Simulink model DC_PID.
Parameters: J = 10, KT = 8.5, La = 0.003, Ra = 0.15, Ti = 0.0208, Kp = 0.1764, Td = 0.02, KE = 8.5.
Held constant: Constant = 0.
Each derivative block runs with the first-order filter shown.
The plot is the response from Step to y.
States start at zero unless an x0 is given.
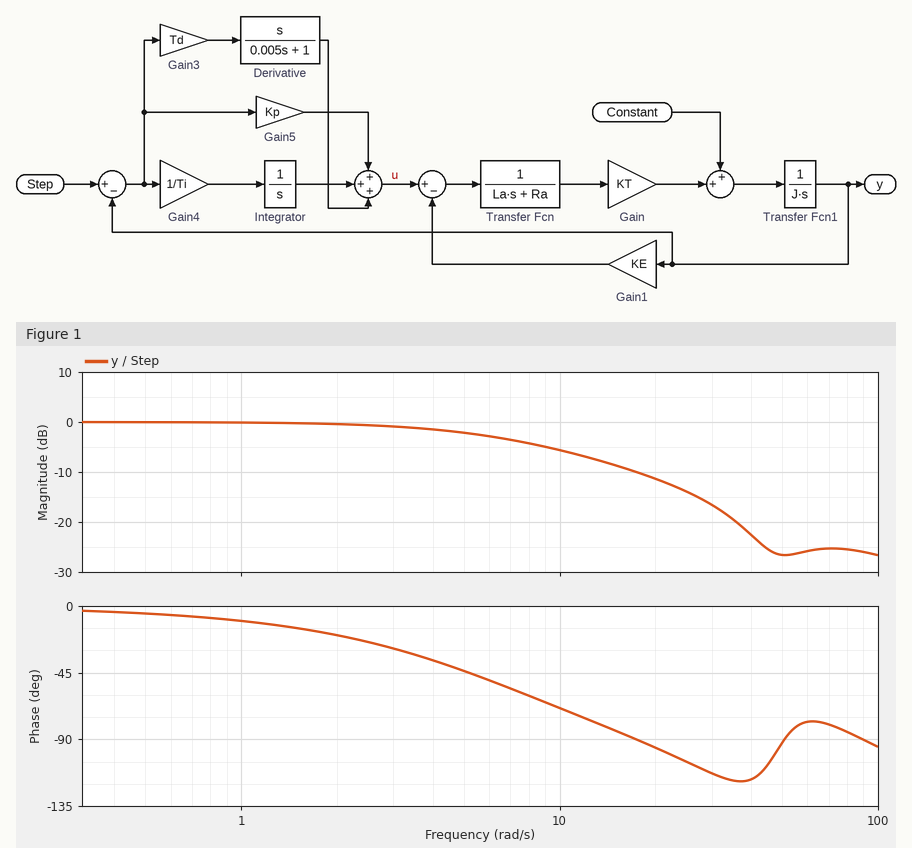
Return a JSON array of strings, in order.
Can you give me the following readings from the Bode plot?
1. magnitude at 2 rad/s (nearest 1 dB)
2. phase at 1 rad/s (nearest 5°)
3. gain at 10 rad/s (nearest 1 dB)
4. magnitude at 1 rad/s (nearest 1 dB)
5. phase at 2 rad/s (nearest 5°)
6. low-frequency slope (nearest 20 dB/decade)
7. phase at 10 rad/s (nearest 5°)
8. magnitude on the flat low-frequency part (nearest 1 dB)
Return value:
["0 dB", "-10°", "-6 dB", "0 dB", "-20°", "0 dB/decade", "-70°", "0 dB"]
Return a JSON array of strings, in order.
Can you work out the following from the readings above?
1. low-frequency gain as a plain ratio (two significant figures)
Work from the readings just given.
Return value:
["1.0"]
